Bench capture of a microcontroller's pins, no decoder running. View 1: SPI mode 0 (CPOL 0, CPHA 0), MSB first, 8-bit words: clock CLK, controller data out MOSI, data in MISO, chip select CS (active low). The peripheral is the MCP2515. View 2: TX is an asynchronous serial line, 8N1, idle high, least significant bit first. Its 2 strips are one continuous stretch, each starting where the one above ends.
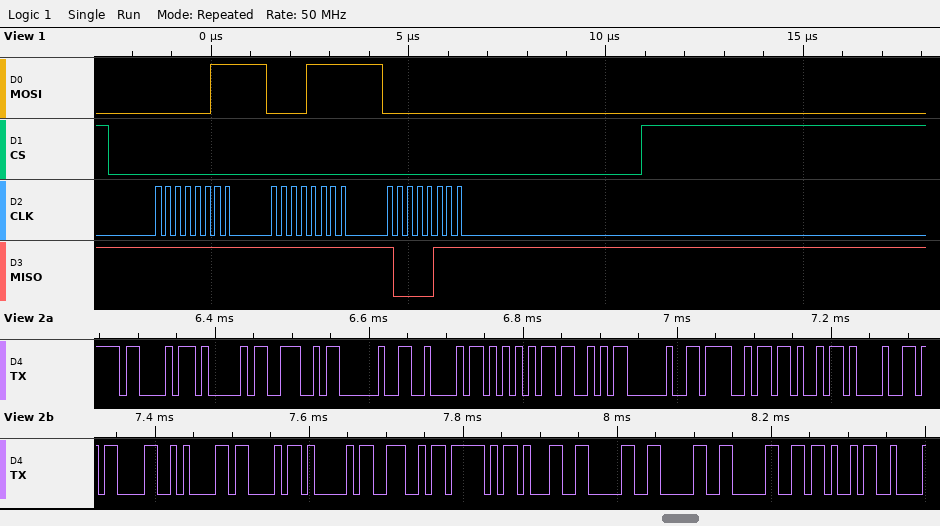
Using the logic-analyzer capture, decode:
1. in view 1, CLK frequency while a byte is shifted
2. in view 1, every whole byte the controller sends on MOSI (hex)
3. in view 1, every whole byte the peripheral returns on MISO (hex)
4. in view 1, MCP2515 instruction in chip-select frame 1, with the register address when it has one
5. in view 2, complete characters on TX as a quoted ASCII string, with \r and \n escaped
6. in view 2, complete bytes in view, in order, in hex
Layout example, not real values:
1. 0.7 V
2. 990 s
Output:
1. 4 MHz
2. 03 0F 00
3. FF FF 87
4. READ 0x0F
5. "CAN BUS OK!\r\nCAN_1000K"
6. 43 41 4E 20 42 55 53 20 4F 4B 21 0D 0A 43 41 4E 5F 31 30 30 30 4B
